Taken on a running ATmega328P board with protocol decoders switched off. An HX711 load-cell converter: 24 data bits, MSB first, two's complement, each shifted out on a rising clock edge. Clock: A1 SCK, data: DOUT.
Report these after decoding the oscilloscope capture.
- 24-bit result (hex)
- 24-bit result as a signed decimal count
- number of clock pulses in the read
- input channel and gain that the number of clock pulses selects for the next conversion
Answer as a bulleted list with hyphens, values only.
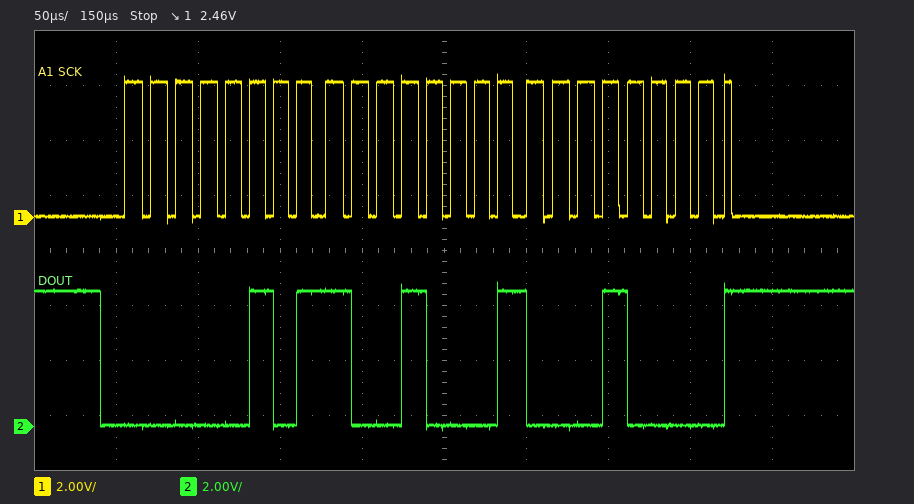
- 0x059110
- 364816
- 25
- channel A, gain 128
